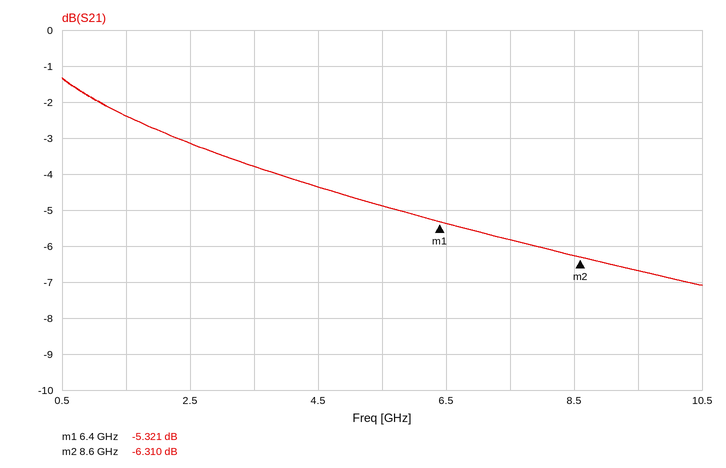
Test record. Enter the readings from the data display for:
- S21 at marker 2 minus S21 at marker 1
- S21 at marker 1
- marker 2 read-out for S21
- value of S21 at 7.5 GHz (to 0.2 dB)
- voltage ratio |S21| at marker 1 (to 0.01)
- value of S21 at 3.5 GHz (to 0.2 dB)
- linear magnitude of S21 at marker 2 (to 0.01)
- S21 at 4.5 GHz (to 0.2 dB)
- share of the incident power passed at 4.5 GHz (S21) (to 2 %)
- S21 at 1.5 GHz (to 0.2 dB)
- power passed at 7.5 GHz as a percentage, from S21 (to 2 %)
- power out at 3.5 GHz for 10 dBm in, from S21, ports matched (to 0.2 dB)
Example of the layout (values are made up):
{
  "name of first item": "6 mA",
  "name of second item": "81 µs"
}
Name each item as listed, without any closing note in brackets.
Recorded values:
{
  "S21 at marker 2 minus S21 at marker 1": "-0.989 dB",
  "S21 at marker 1": "-5.321 dB",
  "marker 2 read-out for S21": "-6.310 dB",
  "value of S21 at 7.5 GHz": "-5.8 dB",
  "voltage ratio |S21| at marker 1": "0.54",
  "value of S21 at 3.5 GHz": "-3.8 dB",
  "linear magnitude of S21 at marker 2": "0.48",
  "S21 at 4.5 GHz": "-4.4 dB",
  "share of the incident power passed at 4.5 GHz (S21)": "36 %",
  "S21 at 1.5 GHz": "-2.4 dB",
  "power passed at 7.5 GHz as a percentage, from S21": "26 %",
  "power out at 3.5 GHz for 10 dBm in, from S21, ports matched": "6.2 dBm"
}
